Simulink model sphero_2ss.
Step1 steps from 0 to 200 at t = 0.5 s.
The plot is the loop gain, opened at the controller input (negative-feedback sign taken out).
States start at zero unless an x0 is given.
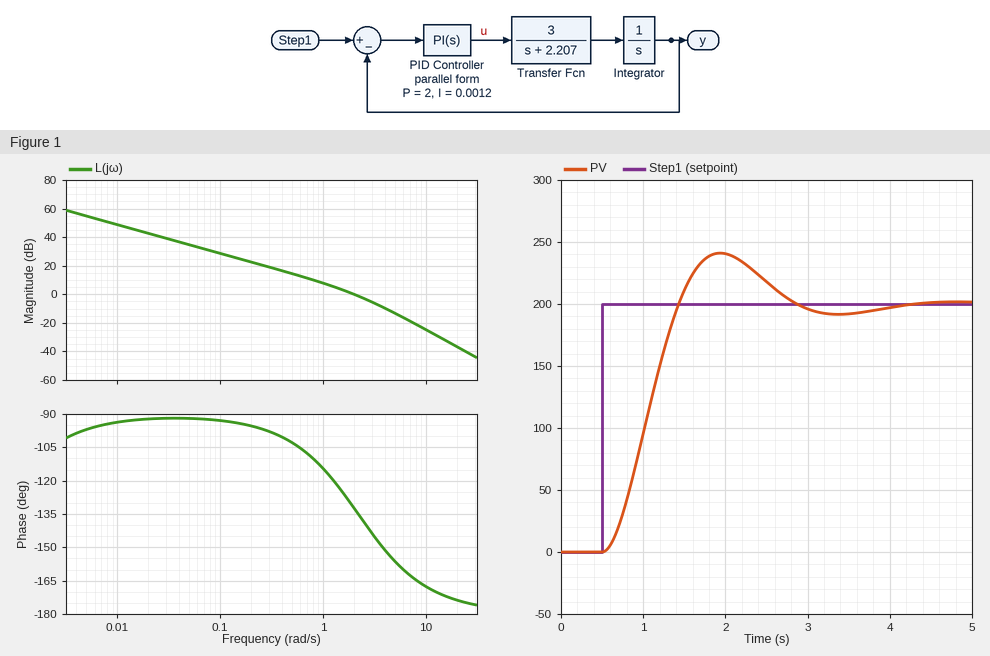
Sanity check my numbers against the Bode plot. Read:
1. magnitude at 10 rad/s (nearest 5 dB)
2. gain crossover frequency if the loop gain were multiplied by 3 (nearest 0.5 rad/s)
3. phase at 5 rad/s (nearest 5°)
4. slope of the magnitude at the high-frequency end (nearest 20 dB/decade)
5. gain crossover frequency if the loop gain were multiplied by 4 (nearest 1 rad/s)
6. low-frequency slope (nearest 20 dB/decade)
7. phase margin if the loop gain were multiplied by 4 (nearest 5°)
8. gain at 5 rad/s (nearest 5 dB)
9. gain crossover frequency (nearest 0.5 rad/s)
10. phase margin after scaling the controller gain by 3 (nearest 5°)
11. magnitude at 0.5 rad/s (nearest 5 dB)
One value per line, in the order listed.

-25 dB
4.0 rad/s
-155°
-40 dB/decade
5 rad/s
-20 dB/decade
25°
-15 dB
2.0 rad/s
30°
15 dB
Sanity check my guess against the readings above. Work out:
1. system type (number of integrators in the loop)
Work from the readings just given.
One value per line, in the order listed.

1
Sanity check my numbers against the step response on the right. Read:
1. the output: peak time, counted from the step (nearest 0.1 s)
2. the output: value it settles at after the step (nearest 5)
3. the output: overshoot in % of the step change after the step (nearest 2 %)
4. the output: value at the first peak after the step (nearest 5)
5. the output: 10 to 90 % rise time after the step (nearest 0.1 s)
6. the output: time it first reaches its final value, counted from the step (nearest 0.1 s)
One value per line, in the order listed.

1.4 s
200
20 %
240
0.6 s
0.9 s
